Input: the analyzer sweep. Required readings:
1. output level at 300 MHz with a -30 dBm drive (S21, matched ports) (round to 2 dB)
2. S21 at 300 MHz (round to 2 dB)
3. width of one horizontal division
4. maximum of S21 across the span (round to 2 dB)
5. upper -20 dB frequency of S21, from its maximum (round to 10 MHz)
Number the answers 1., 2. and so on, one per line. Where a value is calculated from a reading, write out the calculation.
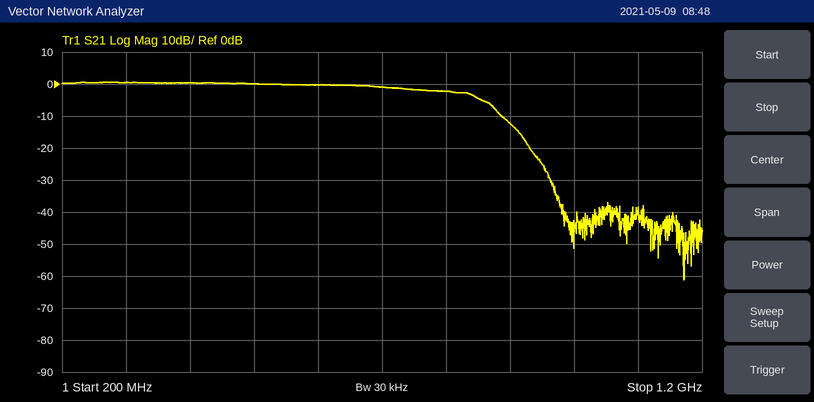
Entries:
1. -30 dBm + (0 dB) = -30 dBm
2. 0 dB
3. 100 MHz
4. 0 dB
5. 930 MHz
